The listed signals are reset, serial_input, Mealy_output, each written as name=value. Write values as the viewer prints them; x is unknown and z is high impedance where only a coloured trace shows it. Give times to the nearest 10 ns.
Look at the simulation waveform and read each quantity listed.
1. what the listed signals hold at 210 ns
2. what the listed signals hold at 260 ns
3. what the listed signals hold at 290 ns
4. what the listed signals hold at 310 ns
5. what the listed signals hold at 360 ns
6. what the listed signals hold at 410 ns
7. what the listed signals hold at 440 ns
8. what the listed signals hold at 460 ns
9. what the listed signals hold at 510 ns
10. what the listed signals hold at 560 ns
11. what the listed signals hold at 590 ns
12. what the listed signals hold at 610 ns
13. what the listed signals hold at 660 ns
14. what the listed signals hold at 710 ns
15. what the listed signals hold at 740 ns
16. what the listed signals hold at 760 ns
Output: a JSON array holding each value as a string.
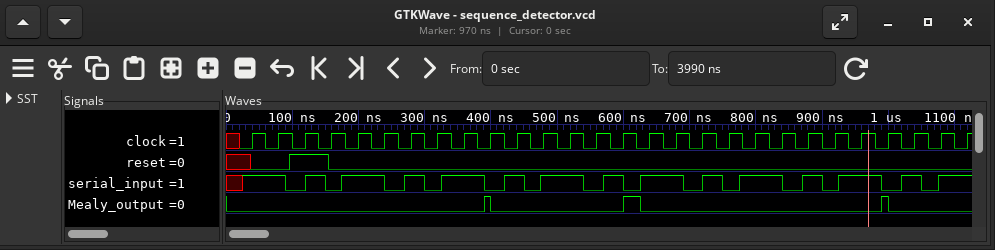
["reset=0, serial_input=1, Mealy_output=0", "reset=0, serial_input=0, Mealy_output=0", "reset=0, serial_input=1, Mealy_output=0", "reset=0, serial_input=0, Mealy_output=0", "reset=0, serial_input=1, Mealy_output=0", "reset=0, serial_input=0, Mealy_output=0", "reset=0, serial_input=1, Mealy_output=0", "reset=0, serial_input=0, Mealy_output=0", "reset=0, serial_input=1, Mealy_output=0", "reset=0, serial_input=0, Mealy_output=0", "reset=0, serial_input=1, Mealy_output=0", "reset=0, serial_input=0, Mealy_output=1", "reset=0, serial_input=1, Mealy_output=0", "reset=0, serial_input=0, Mealy_output=0", "reset=0, serial_input=1, Mealy_output=0", "reset=0, serial_input=0, Mealy_output=0"]
